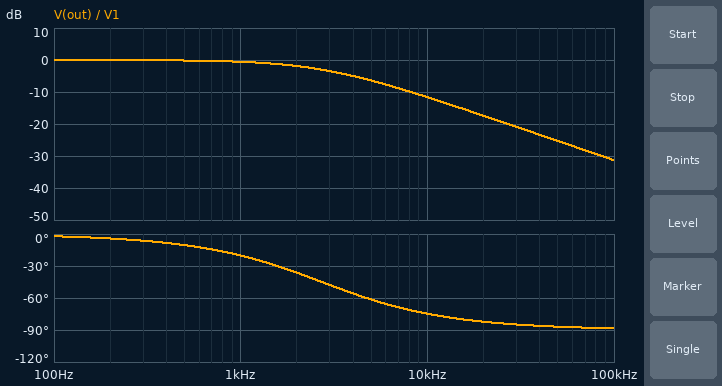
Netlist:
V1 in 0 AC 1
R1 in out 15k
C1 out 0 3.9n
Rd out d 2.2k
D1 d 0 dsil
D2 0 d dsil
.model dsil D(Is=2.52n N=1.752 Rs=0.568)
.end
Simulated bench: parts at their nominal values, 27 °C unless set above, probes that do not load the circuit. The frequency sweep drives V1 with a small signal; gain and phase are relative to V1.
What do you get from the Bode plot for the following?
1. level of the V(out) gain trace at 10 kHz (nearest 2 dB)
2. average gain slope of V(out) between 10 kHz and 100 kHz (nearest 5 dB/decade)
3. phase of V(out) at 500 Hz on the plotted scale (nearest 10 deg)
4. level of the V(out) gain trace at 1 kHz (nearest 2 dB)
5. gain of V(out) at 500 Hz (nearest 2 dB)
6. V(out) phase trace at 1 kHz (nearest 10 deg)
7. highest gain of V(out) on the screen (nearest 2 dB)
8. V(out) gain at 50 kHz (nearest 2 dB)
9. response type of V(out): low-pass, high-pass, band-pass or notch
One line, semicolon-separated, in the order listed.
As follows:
-12 dB; -20 dB/decade; -10 deg; 0 dB; 0 dB; -20 deg; 0 dB; -26 dB; low-pass
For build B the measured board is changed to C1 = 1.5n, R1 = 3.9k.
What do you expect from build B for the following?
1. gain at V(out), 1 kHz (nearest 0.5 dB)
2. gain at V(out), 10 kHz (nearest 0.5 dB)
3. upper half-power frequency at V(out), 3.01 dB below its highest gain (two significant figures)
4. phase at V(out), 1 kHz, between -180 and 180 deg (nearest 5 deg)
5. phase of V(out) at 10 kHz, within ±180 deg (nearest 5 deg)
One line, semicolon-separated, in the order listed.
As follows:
0 dB; -0.5 dB; 27 kHz; 0 deg; -20 deg
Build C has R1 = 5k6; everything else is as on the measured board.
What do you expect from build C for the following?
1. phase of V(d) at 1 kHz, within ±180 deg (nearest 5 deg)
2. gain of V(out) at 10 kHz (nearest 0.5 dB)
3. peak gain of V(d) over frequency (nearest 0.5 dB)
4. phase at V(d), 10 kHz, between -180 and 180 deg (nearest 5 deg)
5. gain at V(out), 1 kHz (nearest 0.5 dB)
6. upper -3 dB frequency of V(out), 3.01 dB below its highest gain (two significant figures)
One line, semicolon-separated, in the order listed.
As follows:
-10 deg; -4.5 dB; 0 dB; -55 deg; 0 dB; 7.3 kHz
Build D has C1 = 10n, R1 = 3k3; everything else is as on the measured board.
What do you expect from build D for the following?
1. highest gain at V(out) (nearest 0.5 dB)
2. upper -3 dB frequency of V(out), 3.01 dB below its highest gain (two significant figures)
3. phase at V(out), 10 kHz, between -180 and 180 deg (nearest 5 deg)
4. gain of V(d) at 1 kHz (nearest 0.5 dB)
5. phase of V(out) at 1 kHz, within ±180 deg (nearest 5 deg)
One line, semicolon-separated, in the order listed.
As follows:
0 dB; 4.8 kHz; -65 deg; 0 dB; -10 deg
